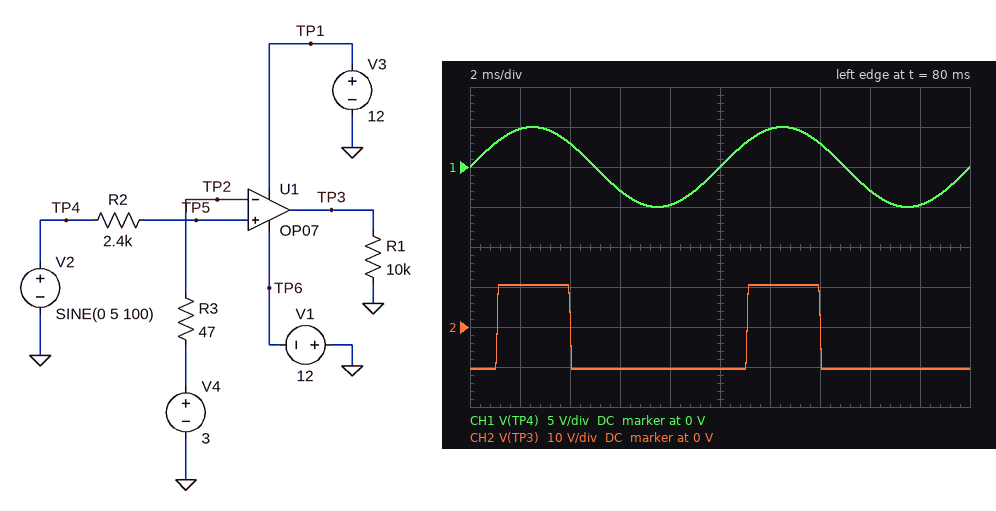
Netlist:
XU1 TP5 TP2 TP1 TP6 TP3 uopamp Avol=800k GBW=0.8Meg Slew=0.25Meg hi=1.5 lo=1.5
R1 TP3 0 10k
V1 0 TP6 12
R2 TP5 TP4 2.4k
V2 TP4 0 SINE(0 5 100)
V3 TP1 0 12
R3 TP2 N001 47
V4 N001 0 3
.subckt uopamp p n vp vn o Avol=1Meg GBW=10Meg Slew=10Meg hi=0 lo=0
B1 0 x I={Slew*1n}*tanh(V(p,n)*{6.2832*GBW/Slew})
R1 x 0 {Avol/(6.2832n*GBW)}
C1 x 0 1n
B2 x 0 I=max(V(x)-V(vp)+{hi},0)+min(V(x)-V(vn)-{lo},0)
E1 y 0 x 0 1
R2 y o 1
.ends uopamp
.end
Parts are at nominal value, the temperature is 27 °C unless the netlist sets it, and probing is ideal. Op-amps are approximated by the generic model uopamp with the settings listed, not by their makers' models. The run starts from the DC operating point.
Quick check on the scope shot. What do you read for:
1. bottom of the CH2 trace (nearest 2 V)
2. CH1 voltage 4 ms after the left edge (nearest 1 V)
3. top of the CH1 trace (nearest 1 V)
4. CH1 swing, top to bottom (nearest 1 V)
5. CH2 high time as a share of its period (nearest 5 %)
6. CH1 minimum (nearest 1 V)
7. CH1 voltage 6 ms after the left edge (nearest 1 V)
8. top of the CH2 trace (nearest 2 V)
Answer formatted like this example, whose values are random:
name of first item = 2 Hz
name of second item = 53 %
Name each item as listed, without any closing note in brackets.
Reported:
bottom of the CH2 trace = -10 V
CH1 voltage 4 ms after the left edge = 3 V
top of the CH1 trace = 5 V
CH1 swing, top to bottom = 10 V
CH2 high time as a share of its period = 30 %
CH1 minimum = -5 V
CH1 voltage 6 ms after the left edge = -3 V
top of the CH2 trace = 10 V
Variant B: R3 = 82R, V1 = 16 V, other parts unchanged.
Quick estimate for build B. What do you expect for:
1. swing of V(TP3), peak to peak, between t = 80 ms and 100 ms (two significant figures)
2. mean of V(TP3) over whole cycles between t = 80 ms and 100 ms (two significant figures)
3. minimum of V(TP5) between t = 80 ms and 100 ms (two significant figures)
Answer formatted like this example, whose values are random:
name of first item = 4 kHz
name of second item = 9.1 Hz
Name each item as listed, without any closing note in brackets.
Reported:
swing of V(TP3), peak to peak, between t = 80 ms and 100 ms = 25 V
mean of V(TP3) over whole cycles between t = 80 ms and 100 ms = -7.1 V
minimum of V(TP5) between t = 80 ms and 100 ms = -5.0 V
